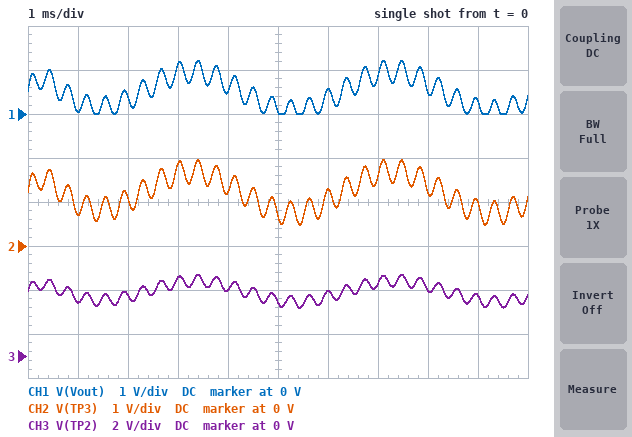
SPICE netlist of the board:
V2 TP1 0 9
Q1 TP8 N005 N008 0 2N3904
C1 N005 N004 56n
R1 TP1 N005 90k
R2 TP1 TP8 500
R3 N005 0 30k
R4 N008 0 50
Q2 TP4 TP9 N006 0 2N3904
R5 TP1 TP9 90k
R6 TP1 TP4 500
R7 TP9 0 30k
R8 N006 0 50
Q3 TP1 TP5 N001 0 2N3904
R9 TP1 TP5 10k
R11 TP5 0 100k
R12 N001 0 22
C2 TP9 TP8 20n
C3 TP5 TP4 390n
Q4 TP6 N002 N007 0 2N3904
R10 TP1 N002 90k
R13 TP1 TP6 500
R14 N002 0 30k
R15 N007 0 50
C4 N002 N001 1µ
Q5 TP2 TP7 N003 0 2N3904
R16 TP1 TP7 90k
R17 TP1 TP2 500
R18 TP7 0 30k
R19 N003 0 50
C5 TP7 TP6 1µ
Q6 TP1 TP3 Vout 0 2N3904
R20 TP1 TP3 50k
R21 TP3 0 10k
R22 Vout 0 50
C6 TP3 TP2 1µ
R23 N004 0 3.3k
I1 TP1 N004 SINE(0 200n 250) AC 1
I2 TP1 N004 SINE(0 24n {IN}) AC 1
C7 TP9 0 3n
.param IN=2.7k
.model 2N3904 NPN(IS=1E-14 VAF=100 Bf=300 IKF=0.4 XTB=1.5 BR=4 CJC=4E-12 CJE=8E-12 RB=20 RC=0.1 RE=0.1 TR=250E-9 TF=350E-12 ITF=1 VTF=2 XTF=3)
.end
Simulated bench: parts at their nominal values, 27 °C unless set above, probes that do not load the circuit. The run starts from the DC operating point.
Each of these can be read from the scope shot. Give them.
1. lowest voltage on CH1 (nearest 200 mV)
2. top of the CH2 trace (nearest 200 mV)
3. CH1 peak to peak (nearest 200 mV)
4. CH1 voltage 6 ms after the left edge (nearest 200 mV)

0 V
2.0 V
1.2 V
600 mV
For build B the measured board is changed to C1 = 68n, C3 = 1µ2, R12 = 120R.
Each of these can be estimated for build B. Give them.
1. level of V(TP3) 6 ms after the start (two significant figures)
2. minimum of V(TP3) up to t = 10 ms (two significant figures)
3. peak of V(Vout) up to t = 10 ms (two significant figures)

1.0 V
280 mV
1.4 V
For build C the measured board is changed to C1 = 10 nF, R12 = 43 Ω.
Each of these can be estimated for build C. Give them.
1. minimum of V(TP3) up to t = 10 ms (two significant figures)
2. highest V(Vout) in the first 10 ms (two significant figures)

830 mV
890 mV
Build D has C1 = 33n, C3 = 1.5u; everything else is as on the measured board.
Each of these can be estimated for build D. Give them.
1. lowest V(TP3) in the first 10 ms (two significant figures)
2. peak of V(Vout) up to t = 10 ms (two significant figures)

580 mV
1.1 V
